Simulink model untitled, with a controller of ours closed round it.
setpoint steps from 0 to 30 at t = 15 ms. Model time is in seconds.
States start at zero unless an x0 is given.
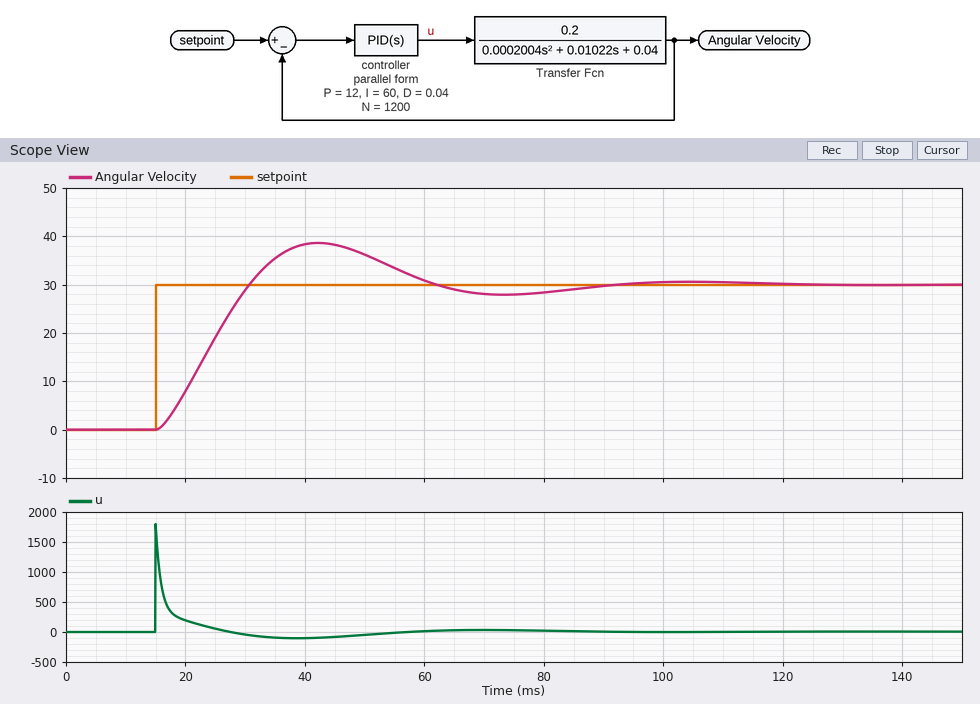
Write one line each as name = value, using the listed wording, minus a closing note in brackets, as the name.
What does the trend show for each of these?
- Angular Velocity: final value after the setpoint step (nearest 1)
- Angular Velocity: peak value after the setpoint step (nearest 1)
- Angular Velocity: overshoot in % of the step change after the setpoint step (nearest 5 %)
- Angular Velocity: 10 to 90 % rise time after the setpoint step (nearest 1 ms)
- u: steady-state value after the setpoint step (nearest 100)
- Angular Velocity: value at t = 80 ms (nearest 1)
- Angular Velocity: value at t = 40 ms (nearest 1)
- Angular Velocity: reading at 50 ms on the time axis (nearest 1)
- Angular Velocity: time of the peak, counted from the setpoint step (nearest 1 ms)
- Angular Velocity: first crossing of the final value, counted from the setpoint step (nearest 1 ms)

Angular Velocity: final value after the setpoint step = 30
Angular Velocity: peak value after the setpoint step = 39
Angular Velocity: overshoot in % of the step change after the setpoint step = 30 %
Angular Velocity: 10 to 90 % rise time after the setpoint step = 11 ms
u: steady-state value after the setpoint step = 0
Angular Velocity: value at t = 80 ms = 28
Angular Velocity: value at t = 40 ms = 38
Angular Velocity: reading at 50 ms on the time axis = 36
Angular Velocity: time of the peak, counted from the setpoint step = 27 ms
Angular Velocity: first crossing of the final value, counted from the setpoint step = 16 ms
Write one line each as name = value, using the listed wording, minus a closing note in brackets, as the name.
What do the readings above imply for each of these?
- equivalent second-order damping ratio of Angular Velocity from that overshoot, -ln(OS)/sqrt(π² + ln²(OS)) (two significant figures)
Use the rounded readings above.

equivalent second-order damping ratio of Angular Velocity from that overshoot, -ln(OS)/sqrt(π² + ln²(OS)) = 0.36
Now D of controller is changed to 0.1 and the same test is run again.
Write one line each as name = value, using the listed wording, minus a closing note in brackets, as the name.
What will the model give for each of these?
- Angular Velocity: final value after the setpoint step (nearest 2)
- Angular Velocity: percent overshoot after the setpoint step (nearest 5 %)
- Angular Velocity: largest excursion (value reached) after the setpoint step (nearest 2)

Angular Velocity: final value after the setpoint step = 30
Angular Velocity: percent overshoot after the setpoint step = 10 %
Angular Velocity: largest excursion (value reached) after the setpoint step = 34
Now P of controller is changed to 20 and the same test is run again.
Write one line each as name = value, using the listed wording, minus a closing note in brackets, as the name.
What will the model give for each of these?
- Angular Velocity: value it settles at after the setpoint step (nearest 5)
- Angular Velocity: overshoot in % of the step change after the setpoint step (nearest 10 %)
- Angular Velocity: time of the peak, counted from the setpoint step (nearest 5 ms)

Angular Velocity: value it settles at after the setpoint step = 30
Angular Velocity: overshoot in % of the step change after the setpoint step = 40 %
Angular Velocity: time of the peak, counted from the setpoint step = 20 ms
